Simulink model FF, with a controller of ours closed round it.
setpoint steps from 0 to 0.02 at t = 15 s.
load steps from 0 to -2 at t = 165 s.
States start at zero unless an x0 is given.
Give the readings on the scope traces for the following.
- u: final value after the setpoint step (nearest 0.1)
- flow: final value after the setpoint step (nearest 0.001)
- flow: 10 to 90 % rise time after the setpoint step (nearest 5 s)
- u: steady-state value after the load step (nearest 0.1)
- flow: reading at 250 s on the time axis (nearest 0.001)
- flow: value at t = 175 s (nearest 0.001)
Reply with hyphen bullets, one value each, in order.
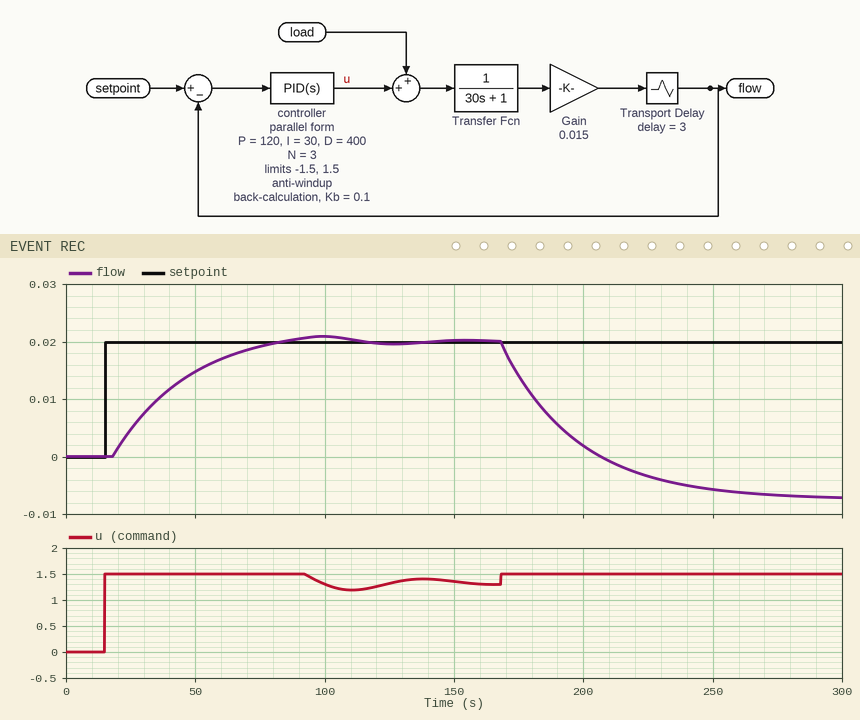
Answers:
- 1.3
- 0.020
- 45 s
- 1.5
- -0.006
- 0.014
